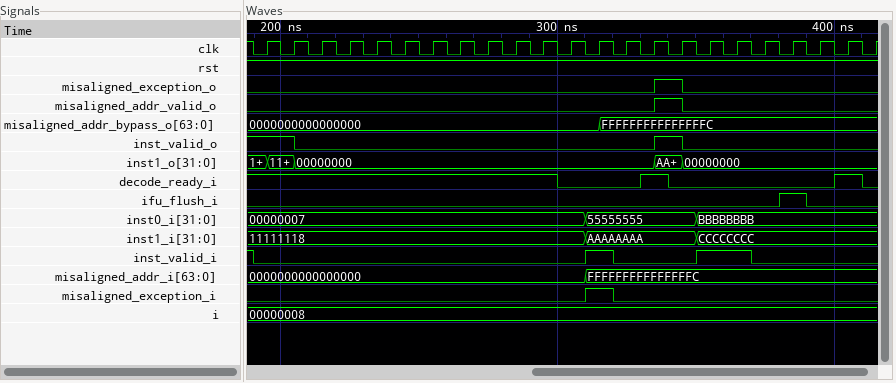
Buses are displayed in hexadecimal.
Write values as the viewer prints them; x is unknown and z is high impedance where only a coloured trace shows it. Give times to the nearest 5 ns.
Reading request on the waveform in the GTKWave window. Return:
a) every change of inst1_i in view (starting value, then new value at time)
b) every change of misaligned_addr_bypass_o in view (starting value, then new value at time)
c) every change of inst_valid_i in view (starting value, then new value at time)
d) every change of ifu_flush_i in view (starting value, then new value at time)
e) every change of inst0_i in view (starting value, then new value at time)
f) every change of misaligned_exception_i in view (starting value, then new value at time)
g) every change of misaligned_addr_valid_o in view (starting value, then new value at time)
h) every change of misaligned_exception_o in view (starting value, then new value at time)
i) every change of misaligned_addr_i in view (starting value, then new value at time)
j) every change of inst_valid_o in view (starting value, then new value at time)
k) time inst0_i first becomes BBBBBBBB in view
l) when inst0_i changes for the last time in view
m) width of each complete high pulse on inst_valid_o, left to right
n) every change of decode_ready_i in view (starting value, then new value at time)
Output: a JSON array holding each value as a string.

["11111118, AAAAAAAA at 310 ns, CCCCCCCC at 350 ns", "0000000000000000, FFFFFFFFFFFFFFFC at 315 ns", "1, 0 at 190 ns, 1 at 310 ns, 0 at 320 ns, 1 at 350 ns, 0 at 370 ns", "0, 1 at 380 ns, 0 at 390 ns", "00000007, 55555555 at 310 ns, BBBBBBBB at 350 ns", "0, 1 at 310 ns, 0 at 320 ns", "0, 1 at 335 ns, 0 at 345 ns", "0, 1 at 335 ns, 0 at 345 ns", "0000000000000000, FFFFFFFFFFFFFFFC at 310 ns", "1, 0 at 205 ns, 1 at 335 ns, 0 at 345 ns", "350 ns", "350 ns", "10 ns", "1, 0 at 300 ns, 1 at 330 ns, 0 at 340 ns, 1 at 400 ns, 0 at 410 ns"]
